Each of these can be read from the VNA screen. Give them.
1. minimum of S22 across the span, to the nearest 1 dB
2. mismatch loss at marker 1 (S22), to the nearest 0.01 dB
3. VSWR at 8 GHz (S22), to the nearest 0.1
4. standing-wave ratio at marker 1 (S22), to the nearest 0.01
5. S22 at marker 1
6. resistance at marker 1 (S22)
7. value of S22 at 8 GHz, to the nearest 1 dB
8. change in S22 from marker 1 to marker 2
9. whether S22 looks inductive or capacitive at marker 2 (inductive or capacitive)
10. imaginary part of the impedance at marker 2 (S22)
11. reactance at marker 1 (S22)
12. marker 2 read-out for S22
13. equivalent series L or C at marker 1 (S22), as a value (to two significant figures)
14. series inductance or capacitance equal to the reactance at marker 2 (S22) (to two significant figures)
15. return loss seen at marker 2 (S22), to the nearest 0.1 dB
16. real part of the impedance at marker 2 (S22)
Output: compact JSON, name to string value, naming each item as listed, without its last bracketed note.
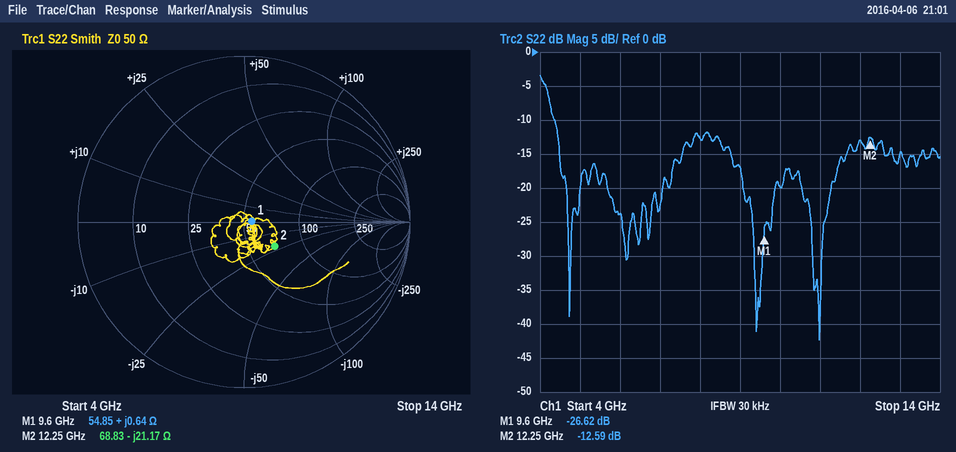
{"minimum of S22 across the span, to the nearest 1 dB": "-42 dB", "mismatch loss at marker 1 (S22), to the nearest 0.01 dB": "0.01 dB", "VSWR at 8 GHz (S22), to the nearest 0.1": "1.6", "standing-wave ratio at marker 1 (S22), to the nearest 0.01": "1.10", "S22 at marker 1": "-26.62 dB", "resistance at marker 1": "54.85 Ω", "value of S22 at 8 GHz, to the nearest 1 dB": "-13 dB", "change in S22 from marker 1 to marker 2": "14.03 dB", "whether S22 looks inductive or capacitive at marker 2": "capacitive", "imaginary part of the impedance at marker 2": "-21.17 Ω", "reactance at marker 1": "+0.64 Ω", "marker 2 read-out for S22": "-12.59 dB", "equivalent series L or C at marker 1 (S22), as a value": "11 pH", "series inductance or capacitance equal to the reactance at marker 2 (S22)": "610 fF", "return loss seen at marker 2 (S22), to the nearest 0.1 dB": "12.6 dB", "real part of the impedance at marker 2": "68.83 Ω"}
